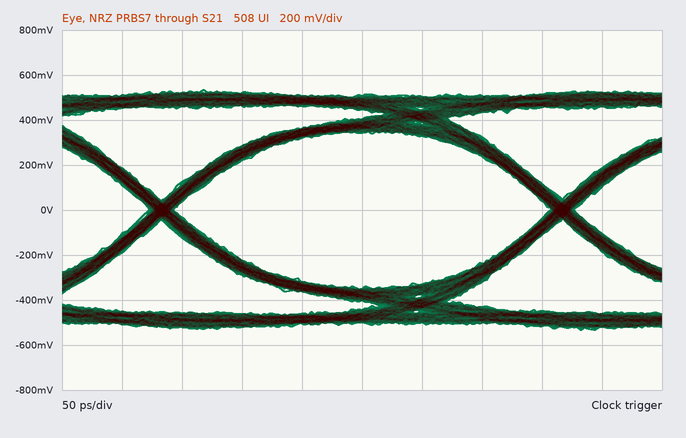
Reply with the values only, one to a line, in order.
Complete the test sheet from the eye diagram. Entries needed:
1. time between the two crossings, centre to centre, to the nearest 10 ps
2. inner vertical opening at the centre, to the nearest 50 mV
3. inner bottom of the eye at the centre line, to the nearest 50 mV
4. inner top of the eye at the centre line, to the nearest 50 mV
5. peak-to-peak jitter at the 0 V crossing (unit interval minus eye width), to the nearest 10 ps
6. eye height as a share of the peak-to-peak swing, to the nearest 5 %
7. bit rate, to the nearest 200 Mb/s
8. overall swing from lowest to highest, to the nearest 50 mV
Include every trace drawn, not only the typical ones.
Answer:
330 ps
700 mV
-350 mV
350 mV
20 ps
65 %
3.0 Gb/s
1.05 V
